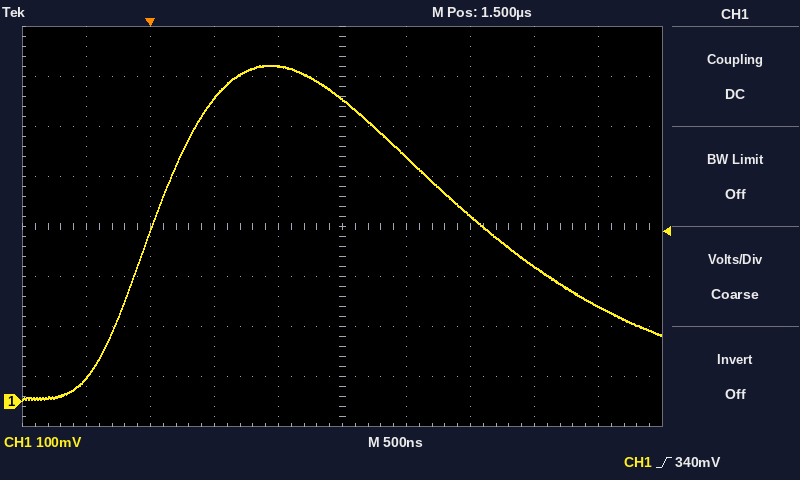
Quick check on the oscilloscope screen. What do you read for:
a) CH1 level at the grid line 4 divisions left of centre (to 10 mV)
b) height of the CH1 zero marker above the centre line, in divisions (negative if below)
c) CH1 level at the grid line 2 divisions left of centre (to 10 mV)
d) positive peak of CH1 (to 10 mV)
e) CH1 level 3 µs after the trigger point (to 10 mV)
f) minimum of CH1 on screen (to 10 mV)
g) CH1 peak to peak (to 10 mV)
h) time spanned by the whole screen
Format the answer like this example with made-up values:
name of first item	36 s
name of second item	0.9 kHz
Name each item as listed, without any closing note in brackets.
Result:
CH1 level at the grid line 4 divisions left of centre	50 mV
height of the CH1 zero marker above the centre line, in divisions	-3.5 div
CH1 level at the grid line 2 divisions left of centre	610 mV
positive peak of CH1	670 mV
CH1 level 3 µs after the trigger point	270 mV
minimum of CH1 on screen	0 mV
CH1 peak to peak	670 mV
time spanned by the whole screen	5 µs
